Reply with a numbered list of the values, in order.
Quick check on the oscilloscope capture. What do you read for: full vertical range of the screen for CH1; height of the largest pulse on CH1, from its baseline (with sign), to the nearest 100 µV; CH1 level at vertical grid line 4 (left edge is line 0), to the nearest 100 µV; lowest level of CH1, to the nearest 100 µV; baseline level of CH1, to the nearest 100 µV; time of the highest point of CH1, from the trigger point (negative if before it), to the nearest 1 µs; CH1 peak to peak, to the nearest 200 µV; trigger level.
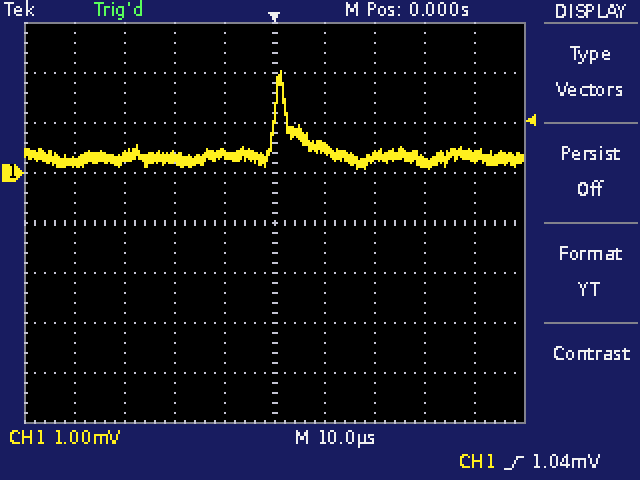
1. 8 mV
2. +1.7 mV
3. 400 µV
4. 100 µV
5. 300 µV
6. +1 µs
7. 2.0 mV
8. 1.04 mV
